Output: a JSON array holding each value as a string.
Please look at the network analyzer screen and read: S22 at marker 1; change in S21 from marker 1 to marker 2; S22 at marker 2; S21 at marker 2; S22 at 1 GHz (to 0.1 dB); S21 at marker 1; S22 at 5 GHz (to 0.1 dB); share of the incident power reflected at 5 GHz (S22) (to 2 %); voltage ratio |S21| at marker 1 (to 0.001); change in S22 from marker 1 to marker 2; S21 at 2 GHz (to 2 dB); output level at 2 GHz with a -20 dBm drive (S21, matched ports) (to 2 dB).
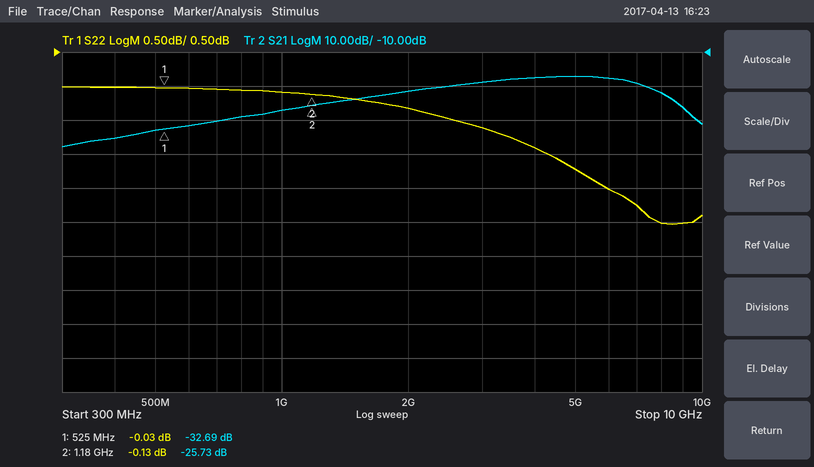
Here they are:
["-0.03 dB", "6.96 dB", "-0.13 dB", "-25.73 dB", "-0.1 dB", "-32.69 dB", "-1.2 dB", "76 %", "0.023", "-0.10 dB", "-22 dB", "-42 dBm"]
